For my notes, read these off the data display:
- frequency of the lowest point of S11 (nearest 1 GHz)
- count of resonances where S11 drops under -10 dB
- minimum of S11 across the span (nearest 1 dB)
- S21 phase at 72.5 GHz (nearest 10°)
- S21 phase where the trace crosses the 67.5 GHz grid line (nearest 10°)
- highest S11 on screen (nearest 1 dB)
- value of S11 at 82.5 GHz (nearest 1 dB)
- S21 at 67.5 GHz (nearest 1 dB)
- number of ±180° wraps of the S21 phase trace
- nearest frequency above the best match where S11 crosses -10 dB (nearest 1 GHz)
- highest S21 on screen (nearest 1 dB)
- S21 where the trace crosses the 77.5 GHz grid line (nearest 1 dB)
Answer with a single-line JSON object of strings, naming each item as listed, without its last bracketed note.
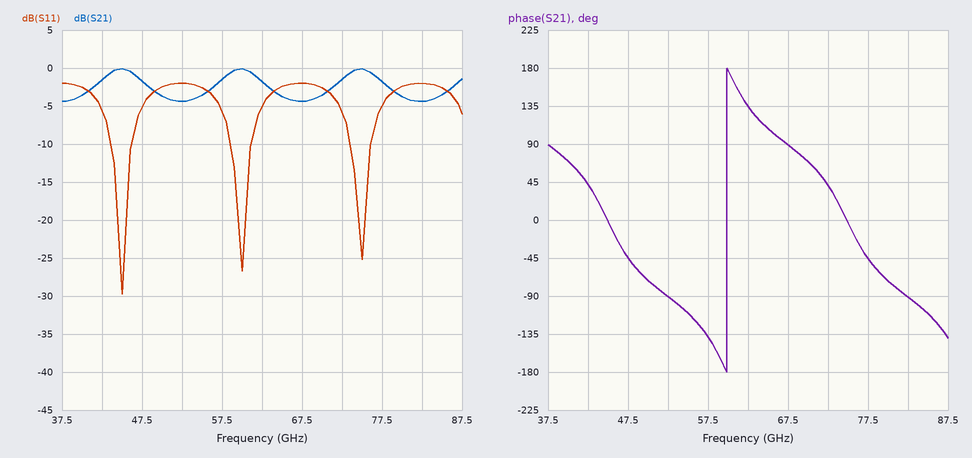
{"frequency of the lowest point of S11": "45 GHz", "count of resonances where S11 drops under -10 dB": "3", "minimum of S11 across the span": "-30 dB", "S21 phase at 72.5 GHz": "40°", "S21 phase where the trace crosses the 67.5 GHz grid line": "90°", "highest S11 on screen": "-2 dB", "value of S11 at 82.5 GHz": "-2 dB", "S21 at 67.5 GHz": "-4 dB", "number of ±180° wraps of the S21 phase trace": "1", "nearest frequency above the best match where S11 crosses -10 dB": "46 GHz", "highest S21 on screen": "0 dB", "S21 where the trace crosses the 77.5 GHz grid line": "-2 dB"}
